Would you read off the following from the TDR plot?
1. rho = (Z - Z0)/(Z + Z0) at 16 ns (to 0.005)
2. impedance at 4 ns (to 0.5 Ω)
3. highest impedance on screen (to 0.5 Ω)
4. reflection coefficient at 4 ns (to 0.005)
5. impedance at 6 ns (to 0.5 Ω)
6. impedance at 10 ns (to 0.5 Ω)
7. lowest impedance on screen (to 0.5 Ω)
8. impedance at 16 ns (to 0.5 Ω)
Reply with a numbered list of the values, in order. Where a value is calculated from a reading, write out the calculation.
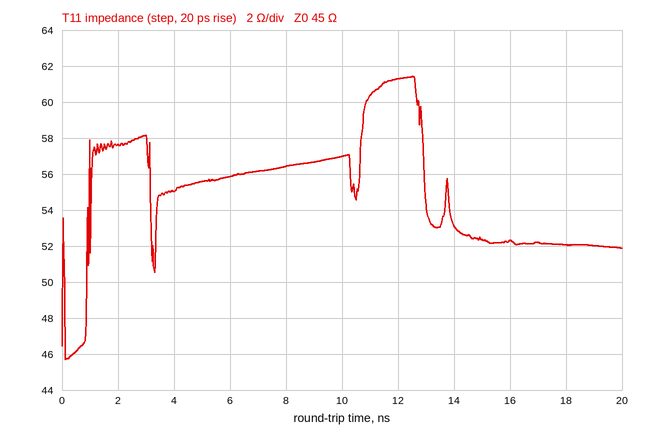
1. (52.5 − 45)/(52.5 + 45) ≈ +0.0769, so +0.075 to the nearest 0.005
2. 55.0 Ω
3. 61.5 Ω
4. (55 − 45)/(55 + 45) ≈ +0.100
5. 56.0 Ω
6. 57.0 Ω
7. 45.5 Ω
8. 52.5 Ω
